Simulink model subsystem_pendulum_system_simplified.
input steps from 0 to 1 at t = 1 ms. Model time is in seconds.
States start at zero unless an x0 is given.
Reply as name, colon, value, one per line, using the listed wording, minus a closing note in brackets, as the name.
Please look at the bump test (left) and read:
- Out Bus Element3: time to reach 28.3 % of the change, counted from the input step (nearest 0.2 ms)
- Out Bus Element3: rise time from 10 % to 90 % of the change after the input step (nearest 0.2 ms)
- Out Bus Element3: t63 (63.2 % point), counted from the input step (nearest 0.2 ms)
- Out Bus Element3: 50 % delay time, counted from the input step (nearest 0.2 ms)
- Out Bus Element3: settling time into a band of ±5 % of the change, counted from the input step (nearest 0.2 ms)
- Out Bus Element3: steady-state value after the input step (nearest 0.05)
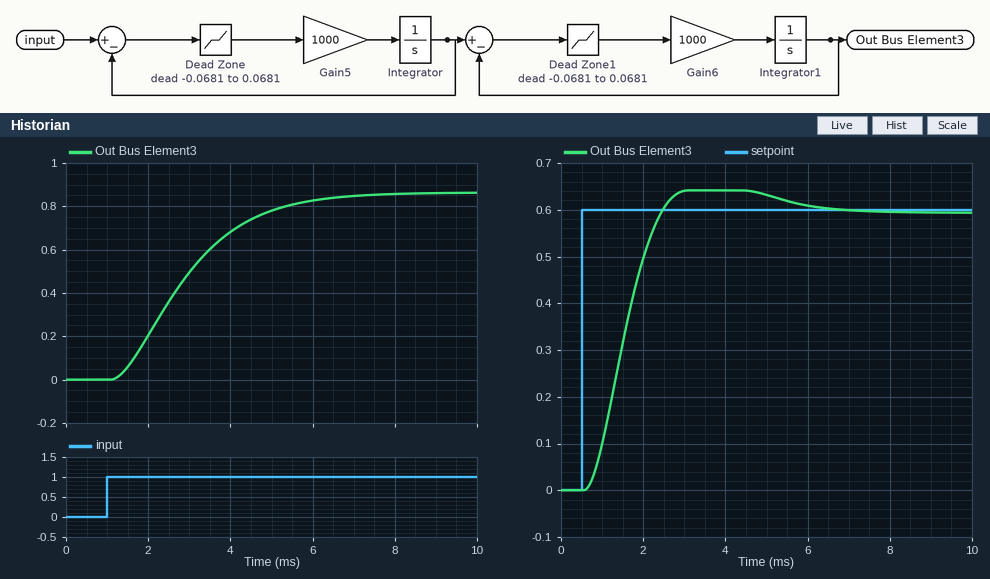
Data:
Out Bus Element3: time to reach 28.3 % of the change, counted from the input step: 1.2 ms
Out Bus Element3: rise time from 10 % to 90 % of the change after the input step: 3.4 ms
Out Bus Element3: t63 (63.2 % point), counted from the input step: 2.2 ms
Out Bus Element3: 50 % delay time, counted from the input step: 1.8 ms
Out Bus Element3: settling time into a band of ±5 % of the change, counted from the input step: 4.8 ms
Out Bus Element3: steady-state value after the input step: 0.85
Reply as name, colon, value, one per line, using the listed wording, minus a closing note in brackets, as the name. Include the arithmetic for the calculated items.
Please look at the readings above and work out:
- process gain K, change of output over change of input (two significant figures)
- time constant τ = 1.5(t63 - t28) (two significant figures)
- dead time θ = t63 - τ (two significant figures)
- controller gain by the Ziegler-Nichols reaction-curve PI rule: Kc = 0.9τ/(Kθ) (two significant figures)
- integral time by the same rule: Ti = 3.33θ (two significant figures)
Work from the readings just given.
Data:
process gain K, change of output over change of input: (0.85 - 0) / 1 = 0.85
time constant τ = 1.5(t63 - t28): 1.5 × (2.2 - 1.2) = 1.5 ms
dead time θ = t63 - τ: 2.2 - 1.5 = 0.70 ms
controller gain by the Ziegler-Nichols reaction-curve PI rule: Kc = 0.9τ/(Kθ): 0.9 × 1.5 / (0.85 × 0.7) = 2.3
integral time by the same rule: Ti = 3.33θ: 3.33 × 0.7 = 2.3 ms
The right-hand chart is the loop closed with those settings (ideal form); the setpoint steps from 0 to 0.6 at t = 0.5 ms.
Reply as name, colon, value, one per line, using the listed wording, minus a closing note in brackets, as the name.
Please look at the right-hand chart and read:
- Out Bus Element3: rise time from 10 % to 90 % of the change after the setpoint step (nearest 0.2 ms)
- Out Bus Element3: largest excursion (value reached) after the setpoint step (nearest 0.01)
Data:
Out Bus Element3: rise time from 10 % to 90 % of the change after the setpoint step: 1.2 ms
Out Bus Element3: largest excursion (value reached) after the setpoint step: 0.64
